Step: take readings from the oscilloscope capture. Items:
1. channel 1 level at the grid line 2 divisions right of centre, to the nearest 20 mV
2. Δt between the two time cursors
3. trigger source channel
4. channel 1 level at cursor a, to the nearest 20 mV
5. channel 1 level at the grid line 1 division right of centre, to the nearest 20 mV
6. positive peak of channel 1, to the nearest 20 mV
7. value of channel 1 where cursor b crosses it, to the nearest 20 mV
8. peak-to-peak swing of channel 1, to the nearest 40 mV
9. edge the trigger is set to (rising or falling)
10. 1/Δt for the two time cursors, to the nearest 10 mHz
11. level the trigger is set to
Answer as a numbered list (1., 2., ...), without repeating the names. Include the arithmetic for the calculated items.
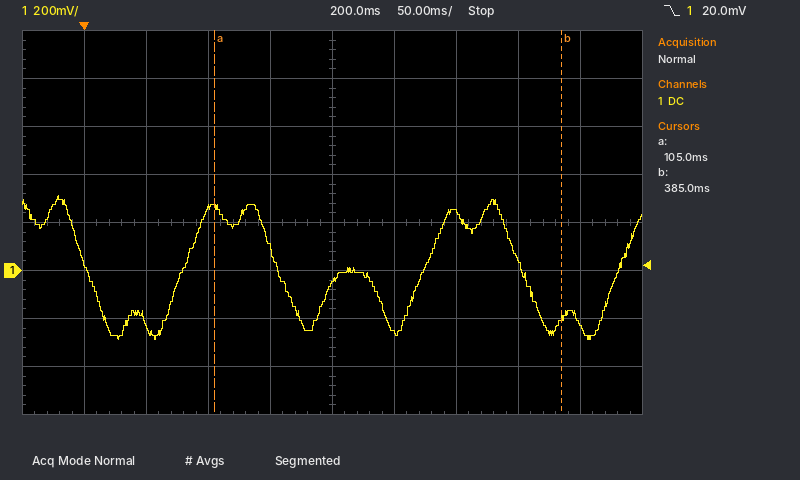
1. 240 mV
2. 385 ms − (105 ms) = 280 ms
3. channel 1
4. 260 mV
5. -260 mV
6. 320 mV
7. -200 mV
8. 600 mV
9. falling
10. 1 / 280 ms ≈ 3.57 Hz
11. 20.0 mV
